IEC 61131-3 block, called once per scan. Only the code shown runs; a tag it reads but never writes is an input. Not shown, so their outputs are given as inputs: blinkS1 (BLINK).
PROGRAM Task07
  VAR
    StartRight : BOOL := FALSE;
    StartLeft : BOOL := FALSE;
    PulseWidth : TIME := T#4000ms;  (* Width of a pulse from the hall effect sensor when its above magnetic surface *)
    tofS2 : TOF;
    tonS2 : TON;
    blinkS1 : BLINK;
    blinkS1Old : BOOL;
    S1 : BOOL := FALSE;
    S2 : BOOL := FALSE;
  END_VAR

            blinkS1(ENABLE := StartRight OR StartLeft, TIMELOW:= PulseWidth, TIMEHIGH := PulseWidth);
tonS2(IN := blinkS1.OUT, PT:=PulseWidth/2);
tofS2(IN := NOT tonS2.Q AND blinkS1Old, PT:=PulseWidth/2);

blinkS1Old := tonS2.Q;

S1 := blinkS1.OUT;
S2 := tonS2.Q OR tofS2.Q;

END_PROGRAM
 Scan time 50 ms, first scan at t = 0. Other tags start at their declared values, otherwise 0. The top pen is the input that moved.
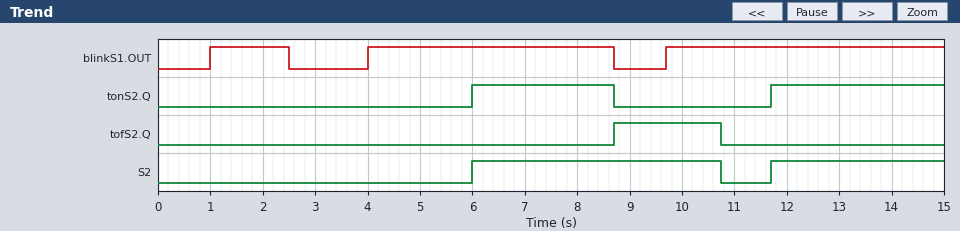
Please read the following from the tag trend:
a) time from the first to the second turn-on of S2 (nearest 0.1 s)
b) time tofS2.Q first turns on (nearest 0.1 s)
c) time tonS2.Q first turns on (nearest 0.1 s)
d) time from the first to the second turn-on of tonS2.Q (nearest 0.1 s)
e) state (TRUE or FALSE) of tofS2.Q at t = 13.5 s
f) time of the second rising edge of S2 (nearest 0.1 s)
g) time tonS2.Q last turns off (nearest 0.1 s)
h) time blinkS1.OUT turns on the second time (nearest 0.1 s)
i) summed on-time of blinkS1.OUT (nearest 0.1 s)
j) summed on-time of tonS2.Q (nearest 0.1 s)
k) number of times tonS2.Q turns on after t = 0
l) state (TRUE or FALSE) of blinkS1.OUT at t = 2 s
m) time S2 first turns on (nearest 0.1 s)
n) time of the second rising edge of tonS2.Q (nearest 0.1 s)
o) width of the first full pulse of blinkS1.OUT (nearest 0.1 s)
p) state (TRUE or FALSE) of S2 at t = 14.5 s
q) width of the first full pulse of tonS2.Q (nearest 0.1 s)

5.7 s
8.7 s
6.0 s
5.7 s
FALSE
11.7 s
8.7 s
4.0 s
11.5 s
6.0 s
2
TRUE
6.0 s
11.7 s
1.5 s
TRUE
2.7 s
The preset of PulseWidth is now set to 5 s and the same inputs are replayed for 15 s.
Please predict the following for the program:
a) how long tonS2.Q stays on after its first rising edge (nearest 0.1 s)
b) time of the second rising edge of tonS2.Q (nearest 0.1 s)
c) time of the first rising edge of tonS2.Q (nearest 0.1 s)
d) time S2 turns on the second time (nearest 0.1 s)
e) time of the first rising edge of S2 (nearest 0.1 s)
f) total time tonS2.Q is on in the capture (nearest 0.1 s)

2.2 s
12.2 s
6.5 s
12.2 s
6.5 s
5.0 s
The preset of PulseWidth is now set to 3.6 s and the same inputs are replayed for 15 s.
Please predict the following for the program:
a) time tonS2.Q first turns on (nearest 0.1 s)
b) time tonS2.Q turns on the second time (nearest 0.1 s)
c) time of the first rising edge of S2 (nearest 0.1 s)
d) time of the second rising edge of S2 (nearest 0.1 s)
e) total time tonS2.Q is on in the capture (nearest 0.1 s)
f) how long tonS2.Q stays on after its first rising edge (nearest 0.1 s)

5.8 s
11.5 s
5.8 s
11.5 s
6.4 s
2.9 s
